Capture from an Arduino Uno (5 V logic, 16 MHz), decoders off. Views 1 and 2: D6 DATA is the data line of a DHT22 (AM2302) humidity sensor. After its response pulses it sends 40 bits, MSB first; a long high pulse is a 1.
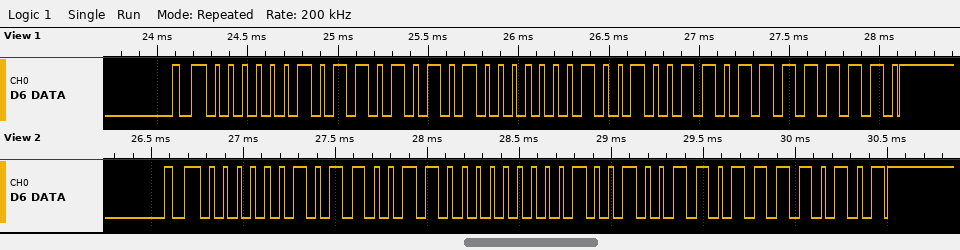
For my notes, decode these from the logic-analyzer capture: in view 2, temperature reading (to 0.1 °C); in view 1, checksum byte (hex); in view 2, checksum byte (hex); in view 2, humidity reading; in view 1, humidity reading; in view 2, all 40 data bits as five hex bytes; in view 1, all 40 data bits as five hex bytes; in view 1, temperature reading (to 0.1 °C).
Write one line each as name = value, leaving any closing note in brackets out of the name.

in view 2, temperature reading = 29.4 °C
in view 1, checksum byte = 0xFE
in view 2, checksum byte = 0xF5
in view 2, humidity reading = 71.6 %
in view 1, humidity reading = 72.5 %
in view 2, all 40 data bits as five hex bytes = 02 CC 01 26 F5
in view 1, all 40 data bits as five hex bytes = 02 D5 01 26 FE
in view 1, temperature reading = 29.4 °C
